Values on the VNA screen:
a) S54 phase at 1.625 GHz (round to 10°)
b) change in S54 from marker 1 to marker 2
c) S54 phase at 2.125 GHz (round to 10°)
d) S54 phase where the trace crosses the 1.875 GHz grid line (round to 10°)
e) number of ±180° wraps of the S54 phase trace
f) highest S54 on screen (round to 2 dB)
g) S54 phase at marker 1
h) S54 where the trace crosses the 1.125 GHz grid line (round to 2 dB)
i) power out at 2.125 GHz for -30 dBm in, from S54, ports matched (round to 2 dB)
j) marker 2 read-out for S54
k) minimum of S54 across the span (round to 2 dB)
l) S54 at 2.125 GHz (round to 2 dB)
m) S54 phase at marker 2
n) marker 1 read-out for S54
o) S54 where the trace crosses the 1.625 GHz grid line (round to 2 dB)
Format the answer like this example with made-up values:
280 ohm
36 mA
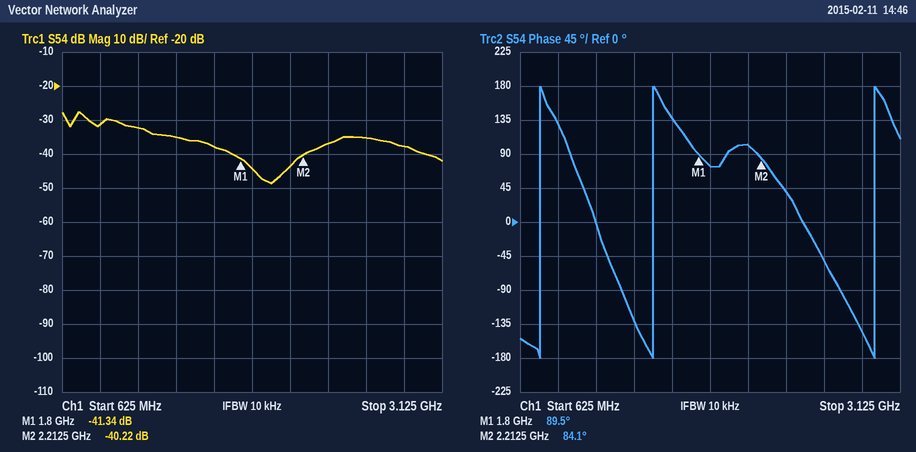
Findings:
140°
1.12 dB
100°
70°
3
-28 dB
89.5°
-32 dB
-74 dBm
-40.22 dB
-48 dB
-44 dB
84.1°
-41.34 dB
-38 dB
